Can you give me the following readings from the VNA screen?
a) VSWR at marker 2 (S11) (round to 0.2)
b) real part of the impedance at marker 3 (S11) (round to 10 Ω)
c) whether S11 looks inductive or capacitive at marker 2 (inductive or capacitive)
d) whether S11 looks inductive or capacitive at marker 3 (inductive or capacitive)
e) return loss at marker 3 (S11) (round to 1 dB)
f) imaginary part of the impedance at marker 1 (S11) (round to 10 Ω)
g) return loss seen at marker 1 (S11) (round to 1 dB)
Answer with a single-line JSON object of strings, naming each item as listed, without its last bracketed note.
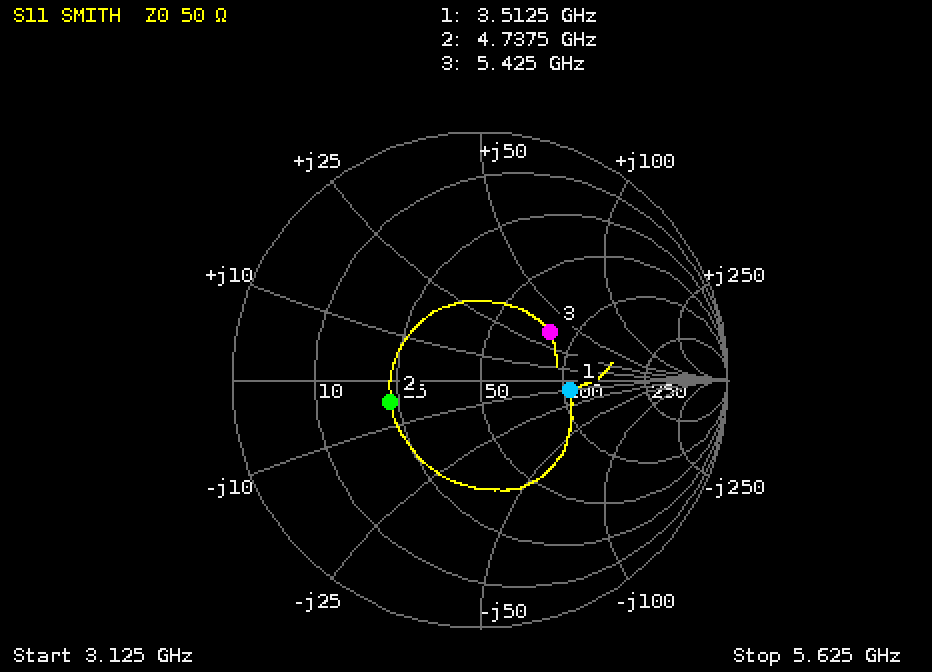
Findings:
{"VSWR at marker 2 (S11)": "2.2", "real part of the impedance at marker 3 (S11)": "80 Ω", "whether S11 looks inductive or capacitive at marker 2": "capacitive", "whether S11 looks inductive or capacitive at marker 3": "inductive", "return loss at marker 3 (S11)": "9 dB", "imaginary part of the impedance at marker 1 (S11)": "-10 Ω", "return loss seen at marker 1 (S11)": "9 dB"}
